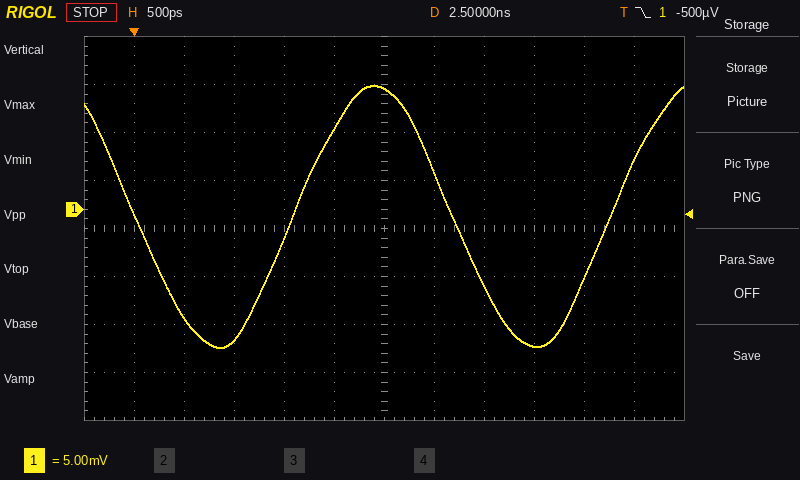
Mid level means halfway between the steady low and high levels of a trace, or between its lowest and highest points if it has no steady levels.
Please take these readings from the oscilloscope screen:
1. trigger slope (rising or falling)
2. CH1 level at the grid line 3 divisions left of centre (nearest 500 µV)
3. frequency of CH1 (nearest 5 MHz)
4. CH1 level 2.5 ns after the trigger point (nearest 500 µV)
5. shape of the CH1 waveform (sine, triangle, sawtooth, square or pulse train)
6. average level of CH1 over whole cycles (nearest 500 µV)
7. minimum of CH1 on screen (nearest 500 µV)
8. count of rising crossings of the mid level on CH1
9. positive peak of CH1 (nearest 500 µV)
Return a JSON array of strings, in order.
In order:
["falling", "-13.5 mV", "315 MHz", "12.5 mV", "sine", "-500 µV", "-14.5 mV", "2", "13.0 mV"]
